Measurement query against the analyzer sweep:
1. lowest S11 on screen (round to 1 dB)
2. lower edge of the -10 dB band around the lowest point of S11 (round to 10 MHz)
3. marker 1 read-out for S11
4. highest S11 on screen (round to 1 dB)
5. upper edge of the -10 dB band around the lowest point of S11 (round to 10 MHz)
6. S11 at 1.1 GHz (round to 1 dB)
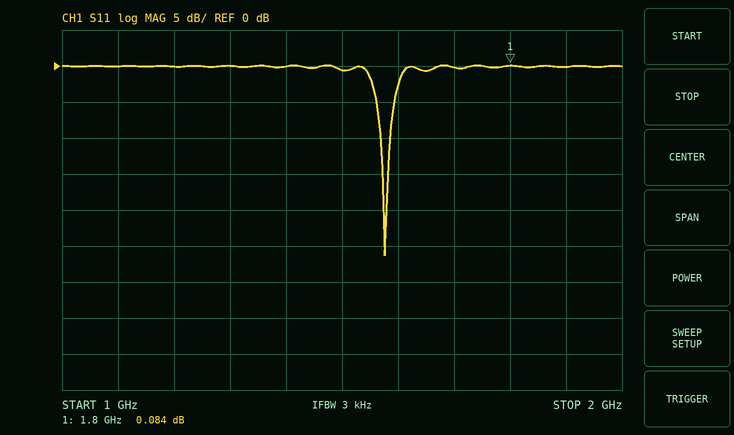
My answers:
-26 dB
1.57 GHz
0.084 dB
0 dB
1.59 GHz
0 dB
